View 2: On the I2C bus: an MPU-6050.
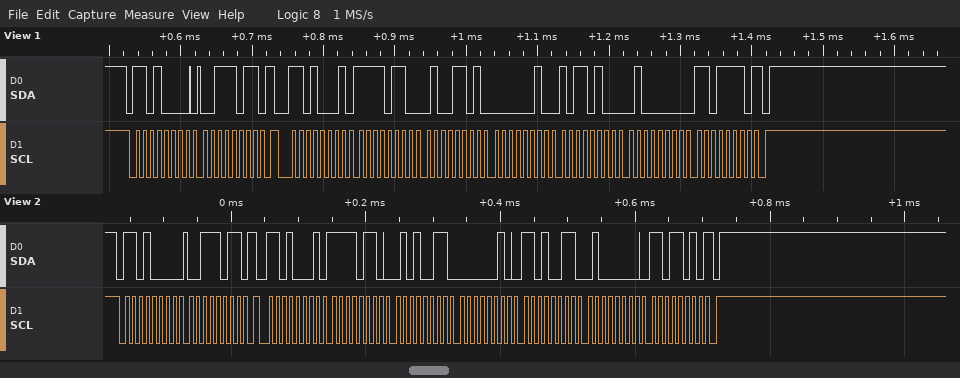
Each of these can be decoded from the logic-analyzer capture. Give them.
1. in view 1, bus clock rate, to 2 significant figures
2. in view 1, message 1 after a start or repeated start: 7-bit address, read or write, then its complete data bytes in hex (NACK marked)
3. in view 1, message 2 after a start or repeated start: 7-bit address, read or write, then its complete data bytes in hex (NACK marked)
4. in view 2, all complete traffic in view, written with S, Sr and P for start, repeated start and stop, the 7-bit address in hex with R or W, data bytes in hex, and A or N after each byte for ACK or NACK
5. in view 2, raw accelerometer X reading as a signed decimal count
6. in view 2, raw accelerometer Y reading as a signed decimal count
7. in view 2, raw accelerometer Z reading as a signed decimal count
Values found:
100 kHz
0x68 write: 3B
0x68 read: F6 4D 02 B4 40 DE NACK
S 68W A 3B A Sr 68R A F6 A 53 A 02 A D3 A 40 A DA N P
-2477
723
16602
